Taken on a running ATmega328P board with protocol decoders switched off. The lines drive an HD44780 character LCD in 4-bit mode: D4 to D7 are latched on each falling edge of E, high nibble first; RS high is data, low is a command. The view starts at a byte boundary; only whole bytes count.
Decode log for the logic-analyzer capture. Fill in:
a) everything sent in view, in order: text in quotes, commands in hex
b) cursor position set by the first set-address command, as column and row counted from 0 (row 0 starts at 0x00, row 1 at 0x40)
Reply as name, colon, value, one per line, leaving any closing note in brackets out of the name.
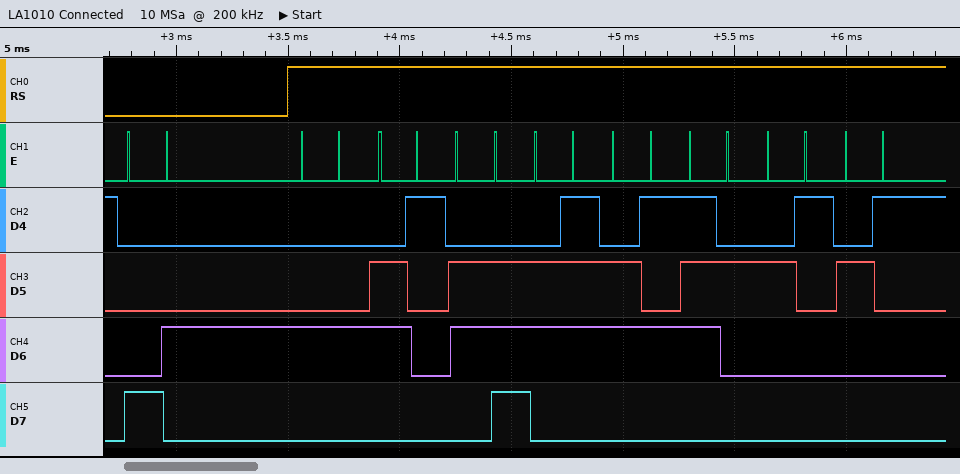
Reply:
everything sent in view, in order: text in quotes, commands in hex: 0x84 "Danger!!"
cursor position set by the first set-address command, as column and row counted from 0: column 4, row 0
